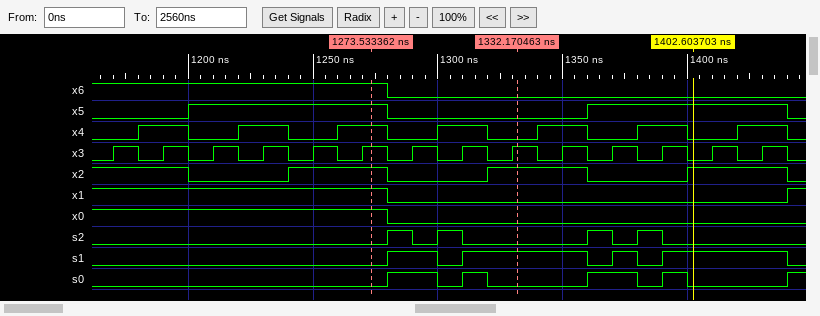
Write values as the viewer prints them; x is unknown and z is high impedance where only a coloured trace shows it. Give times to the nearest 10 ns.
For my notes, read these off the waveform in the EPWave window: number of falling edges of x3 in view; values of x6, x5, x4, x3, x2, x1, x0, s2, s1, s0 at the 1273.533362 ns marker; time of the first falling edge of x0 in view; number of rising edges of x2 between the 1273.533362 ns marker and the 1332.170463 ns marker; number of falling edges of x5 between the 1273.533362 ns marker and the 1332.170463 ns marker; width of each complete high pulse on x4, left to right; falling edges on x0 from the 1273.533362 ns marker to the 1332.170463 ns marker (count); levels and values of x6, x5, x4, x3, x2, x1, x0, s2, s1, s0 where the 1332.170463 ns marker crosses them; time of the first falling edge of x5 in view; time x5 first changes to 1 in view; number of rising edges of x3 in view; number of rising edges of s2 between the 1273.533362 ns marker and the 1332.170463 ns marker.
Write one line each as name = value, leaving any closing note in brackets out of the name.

number of falling edges of x3 in view = 14
values of x6, x5, x4, x3, x2, x1, x0, s2, s1, s0 at the 1273.533362 ns marker = x6=1, x5=1, x4=1, x3=1, x2=1, x1=1, x0=1, s2=0, s1=0, s0=0
time of the first falling edge of x0 in view = 1280 ns
number of rising edges of x2 between the 1273.533362 ns marker and the 1332.170463 ns marker = 1
number of falling edges of x5 between the 1273.533362 ns marker and the 1332.170463 ns marker = 1
width of each complete high pulse on x4, left to right = 20 ns, 20 ns, 20 ns, 20 ns, 20 ns, 20 ns, 20 ns
falling edges on x0 from the 1273.533362 ns marker to the 1332.170463 ns marker = 1
levels and values of x6, x5, x4, x3, x2, x1, x0, s2, s1, s0 where the 1332.170463 ns marker crosses them = x6=0, x5=0, x4=0, x3=1, x2=1, x1=0, x0=0, s2=0, s1=1, s0=0
time of the first falling edge of x5 in view = 1280 ns
time x5 first changes to 1 in view = 1200 ns
number of rising edges of x3 in view = 14
number of rising edges of s2 between the 1273.533362 ns marker and the 1332.170463 ns marker = 2
